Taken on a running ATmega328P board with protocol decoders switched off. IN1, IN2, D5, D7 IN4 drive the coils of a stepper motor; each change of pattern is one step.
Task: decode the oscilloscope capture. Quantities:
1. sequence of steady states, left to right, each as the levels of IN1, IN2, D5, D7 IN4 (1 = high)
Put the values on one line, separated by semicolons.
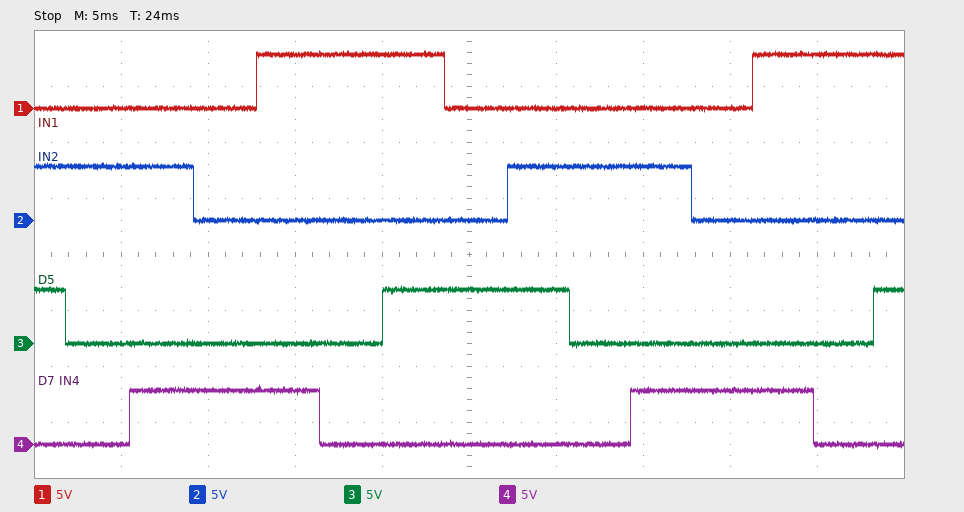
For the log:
0110 0100 0101 0001 1001 1000 1010 0010 0110 0100 0101 0001 1001 1000 1010
